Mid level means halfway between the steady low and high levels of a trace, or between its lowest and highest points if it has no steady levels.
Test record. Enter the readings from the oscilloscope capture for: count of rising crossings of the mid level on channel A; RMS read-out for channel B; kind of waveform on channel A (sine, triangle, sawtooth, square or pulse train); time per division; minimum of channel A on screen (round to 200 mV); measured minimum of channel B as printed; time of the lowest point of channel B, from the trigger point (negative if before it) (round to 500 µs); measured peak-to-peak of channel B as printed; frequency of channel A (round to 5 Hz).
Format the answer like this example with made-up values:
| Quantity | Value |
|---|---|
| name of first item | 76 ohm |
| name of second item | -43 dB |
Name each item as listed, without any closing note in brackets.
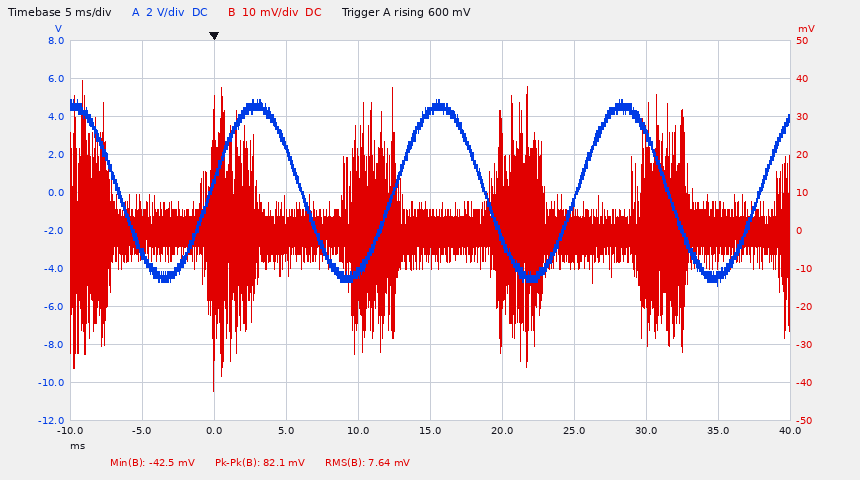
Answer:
| Quantity | Value |
|---|---|
| count of rising crossings of the mid level on channel A | 4 |
| RMS read-out for channel B | 7.64 mV |
| kind of waveform on channel A | sine |
| time per division | 5 ms |
| minimum of channel A on screen | -5.0 V |
| measured minimum of channel B as printed | -42.5 mV |
| time of the lowest point of channel B, from the trigger point (negative if before it) | 0.0 ms |
| measured peak-to-peak of channel B as printed | 82.1 mV |
| frequency of channel A | 80 Hz |
